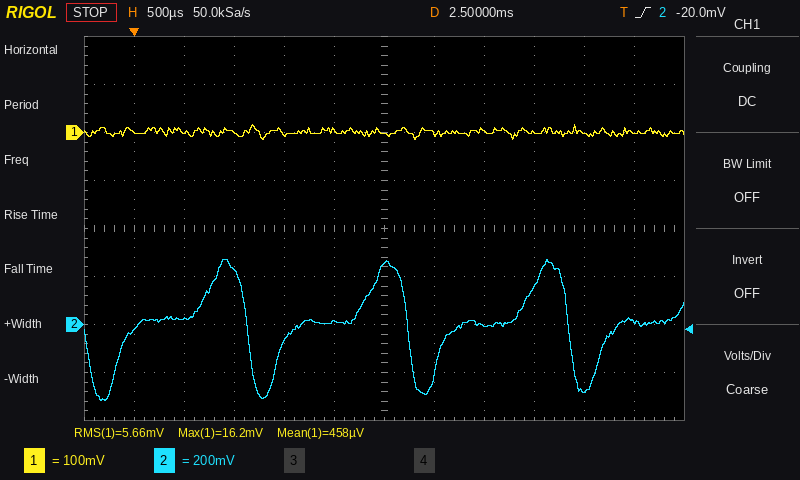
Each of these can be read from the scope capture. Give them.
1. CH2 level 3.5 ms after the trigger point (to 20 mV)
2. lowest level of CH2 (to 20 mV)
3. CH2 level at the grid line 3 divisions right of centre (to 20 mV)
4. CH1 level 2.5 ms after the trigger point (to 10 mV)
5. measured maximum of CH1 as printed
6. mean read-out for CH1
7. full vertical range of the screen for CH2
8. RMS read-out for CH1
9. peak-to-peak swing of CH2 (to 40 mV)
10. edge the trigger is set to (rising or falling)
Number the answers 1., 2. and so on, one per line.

1. 0 mV
2. -320 mV
3. 160 mV
4. 0 mV
5. 16.2 mV
6. 458 µV
7. 1.6 V
8. 5.66 mV
9. 600 mV
10. rising
